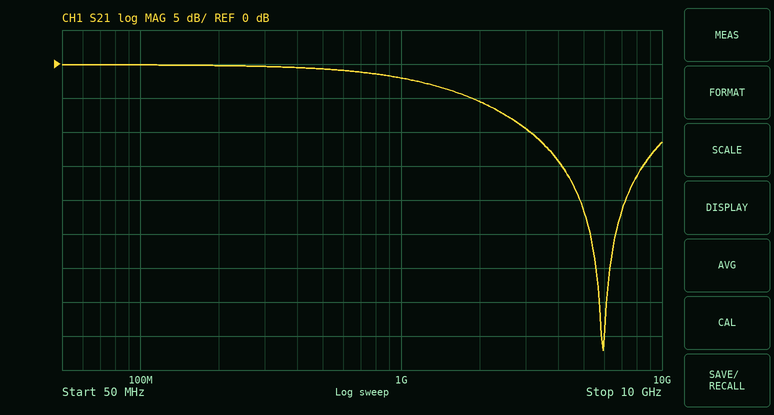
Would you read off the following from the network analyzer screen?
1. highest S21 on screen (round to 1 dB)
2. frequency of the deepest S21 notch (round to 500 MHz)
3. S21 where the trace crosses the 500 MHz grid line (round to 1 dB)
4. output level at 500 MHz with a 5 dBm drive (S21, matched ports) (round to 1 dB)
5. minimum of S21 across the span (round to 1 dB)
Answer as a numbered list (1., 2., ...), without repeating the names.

1. 0 dB
2. 6.0 GHz
3. -1 dB
4. 4 dBm
5. -42 dB
